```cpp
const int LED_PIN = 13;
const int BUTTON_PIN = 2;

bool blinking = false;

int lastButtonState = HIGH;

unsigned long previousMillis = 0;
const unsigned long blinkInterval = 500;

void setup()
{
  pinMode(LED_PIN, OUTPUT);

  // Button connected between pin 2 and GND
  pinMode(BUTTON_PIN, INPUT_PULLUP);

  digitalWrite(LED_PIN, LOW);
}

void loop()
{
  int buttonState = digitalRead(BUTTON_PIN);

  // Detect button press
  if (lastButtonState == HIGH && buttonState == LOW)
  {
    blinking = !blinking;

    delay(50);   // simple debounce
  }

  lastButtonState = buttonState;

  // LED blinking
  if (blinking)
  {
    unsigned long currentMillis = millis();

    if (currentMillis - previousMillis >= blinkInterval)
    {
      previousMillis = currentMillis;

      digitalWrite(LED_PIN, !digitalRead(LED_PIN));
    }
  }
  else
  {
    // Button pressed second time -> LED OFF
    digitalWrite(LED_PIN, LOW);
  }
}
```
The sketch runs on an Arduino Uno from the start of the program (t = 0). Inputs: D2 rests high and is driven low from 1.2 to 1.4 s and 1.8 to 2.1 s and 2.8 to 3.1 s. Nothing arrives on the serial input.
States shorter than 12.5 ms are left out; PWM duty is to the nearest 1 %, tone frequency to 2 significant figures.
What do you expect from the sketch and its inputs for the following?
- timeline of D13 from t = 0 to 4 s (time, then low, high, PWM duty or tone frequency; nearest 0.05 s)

0 s low; 1.25 s high; 1.75 s low; 2.85 s high; 3.35 s low; 3.85 s high
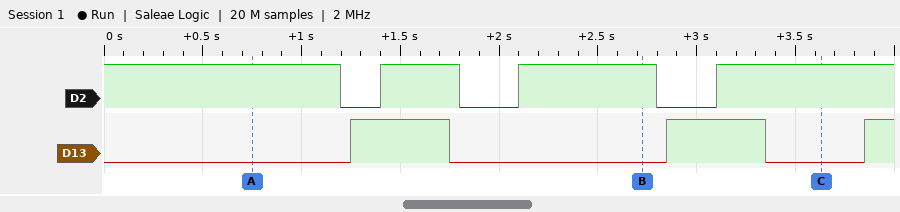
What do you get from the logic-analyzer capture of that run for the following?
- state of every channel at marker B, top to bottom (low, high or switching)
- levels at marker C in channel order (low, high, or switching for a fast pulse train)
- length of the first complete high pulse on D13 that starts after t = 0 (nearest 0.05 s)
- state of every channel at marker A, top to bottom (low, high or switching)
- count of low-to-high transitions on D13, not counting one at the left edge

D2 high, D13 low
D2 high, D13 low
0.50 s
D2 high, D13 low
3
